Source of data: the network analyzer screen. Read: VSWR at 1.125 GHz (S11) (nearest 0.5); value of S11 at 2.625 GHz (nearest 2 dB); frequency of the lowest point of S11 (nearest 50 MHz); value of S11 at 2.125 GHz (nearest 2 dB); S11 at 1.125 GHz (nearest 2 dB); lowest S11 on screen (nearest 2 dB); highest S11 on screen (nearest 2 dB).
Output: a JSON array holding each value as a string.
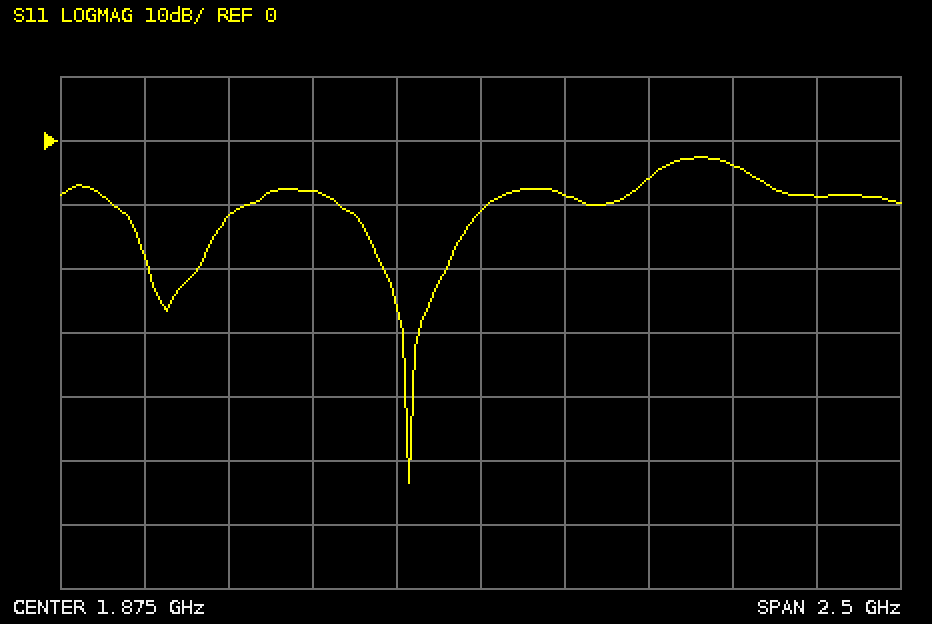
["1.5", "-4 dB", "1.65 GHz", "-8 dB", "-12 dB", "-54 dB", "-2 dB"]
